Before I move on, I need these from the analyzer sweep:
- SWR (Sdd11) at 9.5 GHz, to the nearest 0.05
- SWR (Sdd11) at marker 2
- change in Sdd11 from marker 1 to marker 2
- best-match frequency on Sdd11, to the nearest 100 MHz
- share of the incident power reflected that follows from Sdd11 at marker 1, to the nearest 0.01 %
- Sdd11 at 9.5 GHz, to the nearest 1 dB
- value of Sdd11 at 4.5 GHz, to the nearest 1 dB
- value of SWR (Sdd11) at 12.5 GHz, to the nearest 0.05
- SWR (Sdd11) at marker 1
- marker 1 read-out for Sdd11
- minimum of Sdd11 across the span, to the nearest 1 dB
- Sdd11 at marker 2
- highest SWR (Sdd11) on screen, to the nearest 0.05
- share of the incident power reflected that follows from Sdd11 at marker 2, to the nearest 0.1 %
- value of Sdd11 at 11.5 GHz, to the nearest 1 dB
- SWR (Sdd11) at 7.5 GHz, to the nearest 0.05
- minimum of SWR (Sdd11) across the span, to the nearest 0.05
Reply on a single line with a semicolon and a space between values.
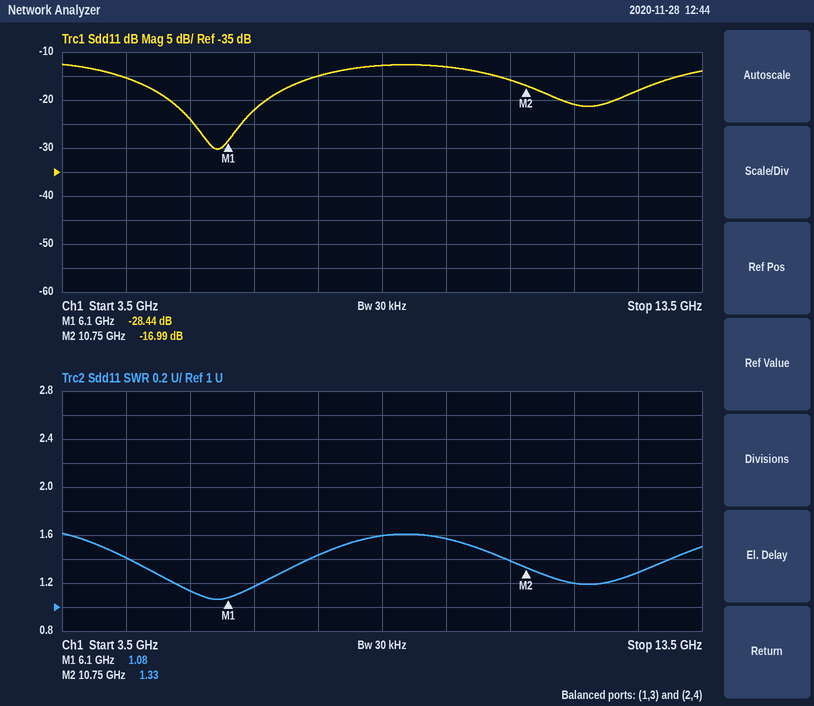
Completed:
1.55; 1.33; 11.45 dB; 5.9 GHz; 0.14 %; -13 dB; -15 dB; 1.30; 1.08; -28.44 dB; -30 dB; -16.99 dB; 1.60; 2.0 %; -21 dB; 1.45; 1.05
